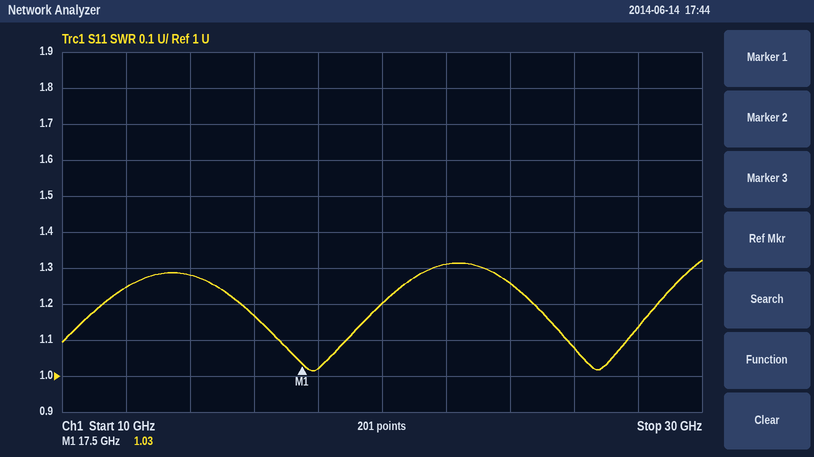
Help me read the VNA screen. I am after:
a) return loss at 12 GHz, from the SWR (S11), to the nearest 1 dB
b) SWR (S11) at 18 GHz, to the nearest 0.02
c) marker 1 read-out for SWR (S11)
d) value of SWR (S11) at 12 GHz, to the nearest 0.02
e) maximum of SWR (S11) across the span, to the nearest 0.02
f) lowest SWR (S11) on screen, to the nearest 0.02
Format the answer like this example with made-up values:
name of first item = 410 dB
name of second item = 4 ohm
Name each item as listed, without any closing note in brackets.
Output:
return loss at 12 GHz, from the SWR (S11), to the nearest 1 dB = 19 dB
SWR (S11) at 18 GHz, to the nearest 0.02 = 1.02
marker 1 read-out for SWR = 1.03
value of SWR (S11) at 12 GHz, to the nearest 0.02 = 1.24
maximum of SWR (S11) across the span, to the nearest 0.02 = 1.32
lowest SWR (S11) on screen, to the nearest 0.02 = 1.02
